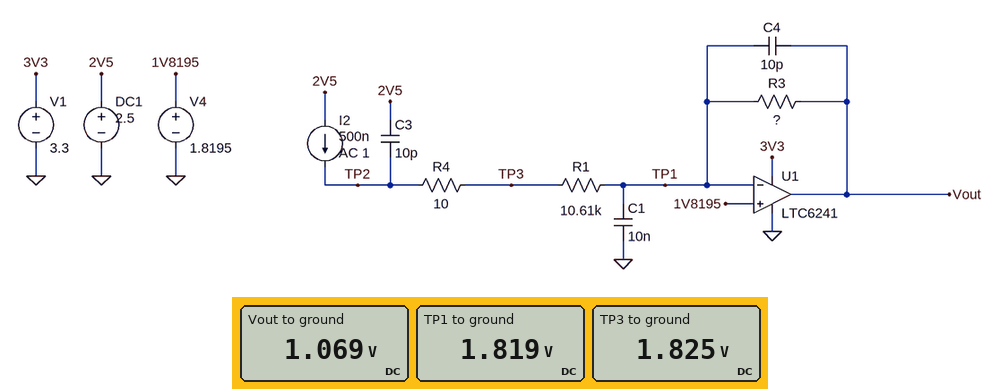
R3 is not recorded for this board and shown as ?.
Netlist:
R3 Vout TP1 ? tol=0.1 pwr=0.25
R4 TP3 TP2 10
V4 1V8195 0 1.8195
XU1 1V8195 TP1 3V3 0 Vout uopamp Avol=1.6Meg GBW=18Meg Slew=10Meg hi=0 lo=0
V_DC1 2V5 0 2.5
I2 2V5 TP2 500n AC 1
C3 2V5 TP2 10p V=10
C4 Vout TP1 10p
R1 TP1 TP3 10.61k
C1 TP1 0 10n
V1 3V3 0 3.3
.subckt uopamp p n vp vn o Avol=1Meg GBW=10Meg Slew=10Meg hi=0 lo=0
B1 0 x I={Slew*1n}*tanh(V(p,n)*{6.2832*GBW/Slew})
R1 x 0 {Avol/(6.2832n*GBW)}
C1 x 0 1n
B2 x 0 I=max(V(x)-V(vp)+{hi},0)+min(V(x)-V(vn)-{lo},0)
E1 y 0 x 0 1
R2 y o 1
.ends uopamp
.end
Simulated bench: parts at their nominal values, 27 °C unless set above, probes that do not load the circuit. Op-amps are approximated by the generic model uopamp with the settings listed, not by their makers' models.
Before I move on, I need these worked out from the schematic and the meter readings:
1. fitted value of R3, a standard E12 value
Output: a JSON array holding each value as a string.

["1.5 MΩ"]
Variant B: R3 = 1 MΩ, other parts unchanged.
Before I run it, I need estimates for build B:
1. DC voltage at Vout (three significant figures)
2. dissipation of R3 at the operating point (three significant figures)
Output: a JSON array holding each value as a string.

["1.32 V", "250 nW"]
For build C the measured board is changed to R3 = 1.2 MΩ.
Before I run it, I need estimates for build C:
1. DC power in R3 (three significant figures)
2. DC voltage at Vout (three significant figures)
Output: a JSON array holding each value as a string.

["300 nW", "1.22 V"]
